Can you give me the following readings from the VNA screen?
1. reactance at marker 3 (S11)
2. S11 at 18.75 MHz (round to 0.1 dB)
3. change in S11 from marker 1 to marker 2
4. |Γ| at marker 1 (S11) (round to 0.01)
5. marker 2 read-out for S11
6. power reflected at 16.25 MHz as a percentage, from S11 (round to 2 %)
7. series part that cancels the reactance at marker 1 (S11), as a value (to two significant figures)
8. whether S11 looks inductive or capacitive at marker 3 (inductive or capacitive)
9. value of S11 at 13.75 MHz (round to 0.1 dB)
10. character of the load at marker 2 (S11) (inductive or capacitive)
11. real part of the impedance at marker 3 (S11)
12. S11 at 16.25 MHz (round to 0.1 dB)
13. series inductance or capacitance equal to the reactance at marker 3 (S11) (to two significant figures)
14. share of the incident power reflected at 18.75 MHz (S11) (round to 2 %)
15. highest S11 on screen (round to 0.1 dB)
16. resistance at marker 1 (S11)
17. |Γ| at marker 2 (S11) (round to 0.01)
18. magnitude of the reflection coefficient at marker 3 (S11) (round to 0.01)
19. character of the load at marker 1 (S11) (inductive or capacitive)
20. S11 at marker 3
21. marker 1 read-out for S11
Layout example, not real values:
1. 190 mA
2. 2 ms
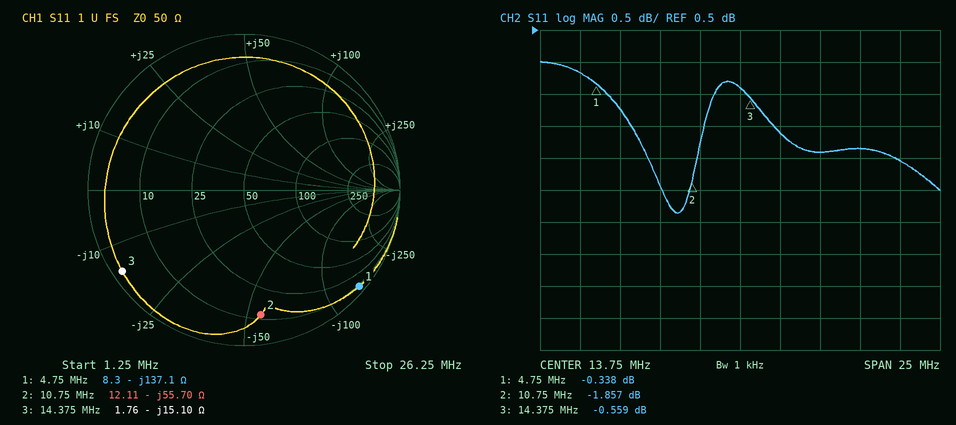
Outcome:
1. -15.10 Ω
2. -1.4 dB
3. -1.519 dB
4. 0.96
5. -1.857 dB
6. 78 %
7. 4.6 µH
8. capacitive
9. -0.4 dB
10. capacitive
11. 1.76 Ω
12. -1.1 dB
13. 730 pF
14. 72 %
15. 0.0 dB
16. 8.3 Ω
17. 0.81
18. 0.94
19. capacitive
20. -0.559 dB
21. -0.338 dB
